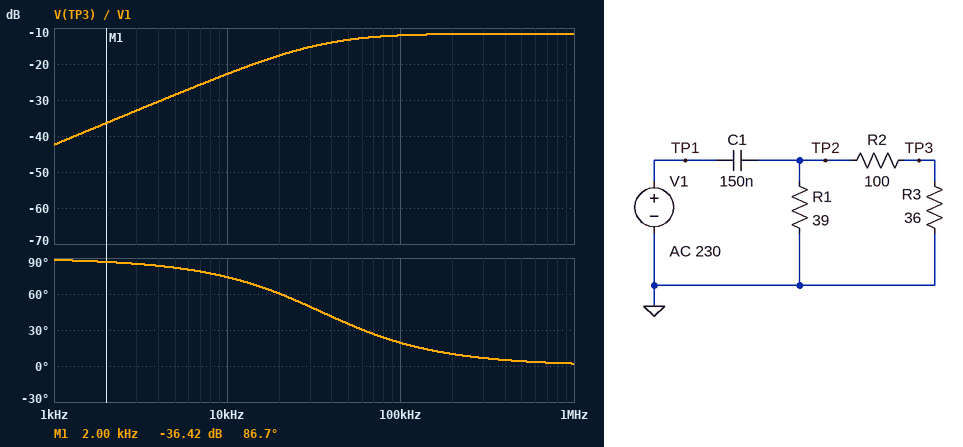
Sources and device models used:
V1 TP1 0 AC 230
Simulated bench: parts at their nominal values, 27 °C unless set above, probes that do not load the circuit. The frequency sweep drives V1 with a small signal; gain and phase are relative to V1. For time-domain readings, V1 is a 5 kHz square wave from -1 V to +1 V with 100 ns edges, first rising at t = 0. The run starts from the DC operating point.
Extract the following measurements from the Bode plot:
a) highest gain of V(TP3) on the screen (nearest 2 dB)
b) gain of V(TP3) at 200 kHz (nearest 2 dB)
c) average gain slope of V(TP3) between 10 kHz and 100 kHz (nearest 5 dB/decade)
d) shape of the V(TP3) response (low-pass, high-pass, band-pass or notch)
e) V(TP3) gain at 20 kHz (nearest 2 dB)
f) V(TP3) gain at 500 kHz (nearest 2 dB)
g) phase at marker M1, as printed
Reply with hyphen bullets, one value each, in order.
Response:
- -12 dB
- -12 dB
- 10 dB/decade
- high-pass
- -18 dB
- -12 dB
- 86.7 deg
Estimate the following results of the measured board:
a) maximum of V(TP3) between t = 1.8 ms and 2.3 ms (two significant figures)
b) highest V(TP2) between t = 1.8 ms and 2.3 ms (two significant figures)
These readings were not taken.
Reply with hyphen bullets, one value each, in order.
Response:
- 520 mV
- 2.0 V
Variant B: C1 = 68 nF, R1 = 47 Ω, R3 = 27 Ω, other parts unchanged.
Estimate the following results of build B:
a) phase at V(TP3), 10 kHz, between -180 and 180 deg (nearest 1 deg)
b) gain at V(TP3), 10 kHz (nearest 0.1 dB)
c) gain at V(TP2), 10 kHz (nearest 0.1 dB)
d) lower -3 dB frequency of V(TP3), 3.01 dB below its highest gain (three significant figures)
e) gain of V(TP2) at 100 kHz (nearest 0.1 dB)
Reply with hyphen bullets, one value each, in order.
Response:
- 82 deg
- -30.2 dB
- -16.8 dB
- 68.2 kHz
- -1.7 dB
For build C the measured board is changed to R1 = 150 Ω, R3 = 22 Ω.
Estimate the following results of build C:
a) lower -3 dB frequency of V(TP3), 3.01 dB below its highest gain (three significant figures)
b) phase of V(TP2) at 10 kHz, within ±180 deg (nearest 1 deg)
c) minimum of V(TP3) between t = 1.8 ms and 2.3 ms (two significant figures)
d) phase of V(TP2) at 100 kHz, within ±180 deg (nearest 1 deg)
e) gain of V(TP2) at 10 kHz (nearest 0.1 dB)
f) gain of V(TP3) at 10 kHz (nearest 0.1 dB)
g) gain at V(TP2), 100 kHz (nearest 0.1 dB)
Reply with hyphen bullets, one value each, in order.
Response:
- 15.8 kHz
- 58 deg
- -360 mV
- 9 deg
- -5.4 dB
- -20.3 dB
- -0.1 dB
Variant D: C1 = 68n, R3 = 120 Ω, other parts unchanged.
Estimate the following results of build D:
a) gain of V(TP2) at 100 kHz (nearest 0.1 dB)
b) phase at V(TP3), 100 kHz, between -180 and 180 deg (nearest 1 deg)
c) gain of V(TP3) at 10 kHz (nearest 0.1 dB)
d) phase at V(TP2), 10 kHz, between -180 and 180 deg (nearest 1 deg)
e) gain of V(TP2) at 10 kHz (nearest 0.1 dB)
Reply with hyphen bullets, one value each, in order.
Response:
- -1.8 dB
- 35 deg
- -22.3 dB
- 82 deg
- -17.1 dB
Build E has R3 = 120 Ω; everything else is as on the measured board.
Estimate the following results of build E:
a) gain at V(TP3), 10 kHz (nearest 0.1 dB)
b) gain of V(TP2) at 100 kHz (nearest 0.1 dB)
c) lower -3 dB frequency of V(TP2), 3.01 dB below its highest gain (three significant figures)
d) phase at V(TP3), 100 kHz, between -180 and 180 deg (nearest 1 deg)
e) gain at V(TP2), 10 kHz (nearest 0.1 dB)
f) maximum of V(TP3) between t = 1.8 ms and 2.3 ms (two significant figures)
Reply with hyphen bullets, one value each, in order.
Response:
- -15.8 dB
- -0.4 dB
- 32.0 kHz
- 18 deg
- -10.5 dB
- 1.1 V
